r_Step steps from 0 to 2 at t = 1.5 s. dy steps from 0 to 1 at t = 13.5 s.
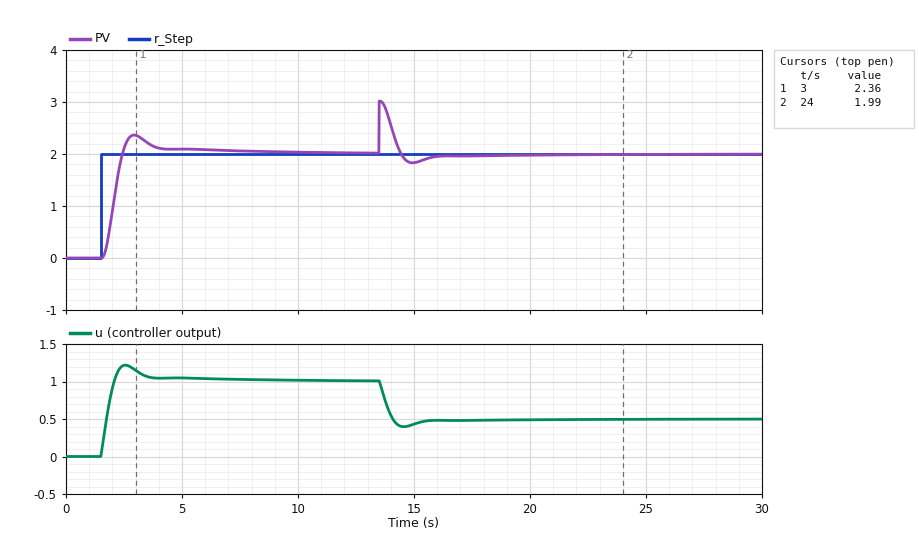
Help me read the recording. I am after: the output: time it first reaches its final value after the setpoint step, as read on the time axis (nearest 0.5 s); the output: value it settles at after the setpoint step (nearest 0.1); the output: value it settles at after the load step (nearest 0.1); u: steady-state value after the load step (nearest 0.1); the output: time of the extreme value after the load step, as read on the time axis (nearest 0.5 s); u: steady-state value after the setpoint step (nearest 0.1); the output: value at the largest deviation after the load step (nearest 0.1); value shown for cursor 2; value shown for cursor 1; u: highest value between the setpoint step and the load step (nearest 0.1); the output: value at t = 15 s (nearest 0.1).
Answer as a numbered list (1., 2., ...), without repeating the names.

1. 2.5 s
2. 2.0
3. 2.0
4. 0.5
5. 13.5 s
6. 1.0
7. 3.0
8. 1.99
9. 2.36
10. 1.2
11. 1.8
